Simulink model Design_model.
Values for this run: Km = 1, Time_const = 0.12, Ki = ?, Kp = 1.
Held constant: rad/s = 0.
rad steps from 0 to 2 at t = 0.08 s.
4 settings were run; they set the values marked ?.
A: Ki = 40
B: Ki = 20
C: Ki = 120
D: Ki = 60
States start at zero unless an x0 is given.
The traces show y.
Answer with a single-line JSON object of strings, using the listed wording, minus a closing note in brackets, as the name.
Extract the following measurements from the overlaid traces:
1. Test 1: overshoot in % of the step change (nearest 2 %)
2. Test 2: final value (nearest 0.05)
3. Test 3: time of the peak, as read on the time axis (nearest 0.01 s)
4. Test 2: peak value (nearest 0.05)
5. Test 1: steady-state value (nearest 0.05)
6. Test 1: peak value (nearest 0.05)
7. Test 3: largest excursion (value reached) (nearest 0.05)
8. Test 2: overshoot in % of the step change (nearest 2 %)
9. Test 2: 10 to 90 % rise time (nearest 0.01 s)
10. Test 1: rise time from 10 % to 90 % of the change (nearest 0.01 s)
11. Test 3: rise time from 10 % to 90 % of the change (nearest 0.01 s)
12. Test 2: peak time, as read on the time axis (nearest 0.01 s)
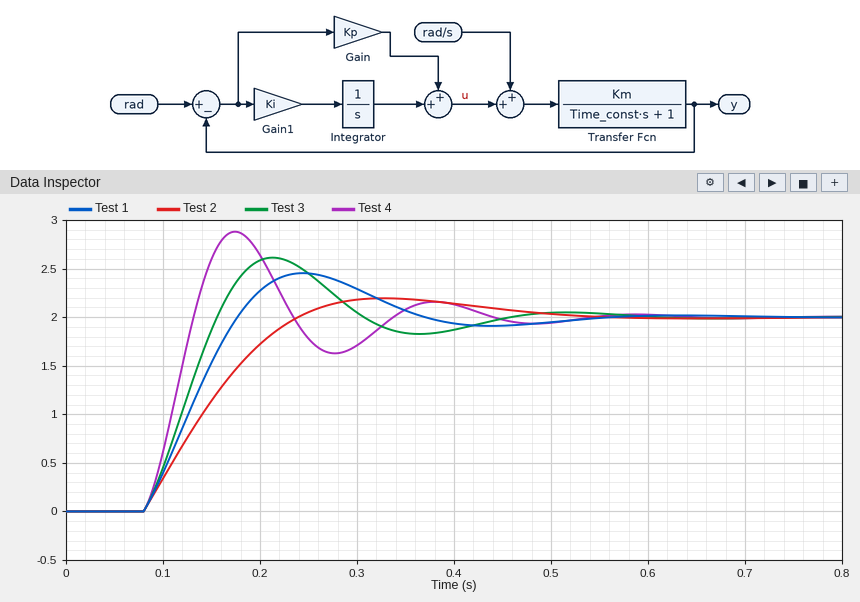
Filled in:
{"Test 1: overshoot in % of the step change": "22 %", "Test 2: final value": "2.00", "Test 3: time of the peak, as read on the time axis": "0.21 s", "Test 2: peak value": "2.20", "Test 1: steady-state value": "2.00", "Test 1: peak value": "2.45", "Test 3: largest excursion (value reached)": "2.60", "Test 2: overshoot in % of the step change": "10 %", "Test 2: 10 to 90 % rise time": "0.12 s", "Test 1: rise time from 10 % to 90 % of the change": "0.07 s", "Test 3: rise time from 10 % to 90 % of the change": "0.06 s", "Test 2: peak time, as read on the time axis": "0.33 s"}
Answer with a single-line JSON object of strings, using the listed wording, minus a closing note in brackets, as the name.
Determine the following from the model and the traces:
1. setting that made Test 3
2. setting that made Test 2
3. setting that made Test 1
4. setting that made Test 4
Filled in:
{"setting that made Test 3": "D", "setting that made Test 2": "B", "setting that made Test 1": "A", "setting that made Test 4": "C"}
